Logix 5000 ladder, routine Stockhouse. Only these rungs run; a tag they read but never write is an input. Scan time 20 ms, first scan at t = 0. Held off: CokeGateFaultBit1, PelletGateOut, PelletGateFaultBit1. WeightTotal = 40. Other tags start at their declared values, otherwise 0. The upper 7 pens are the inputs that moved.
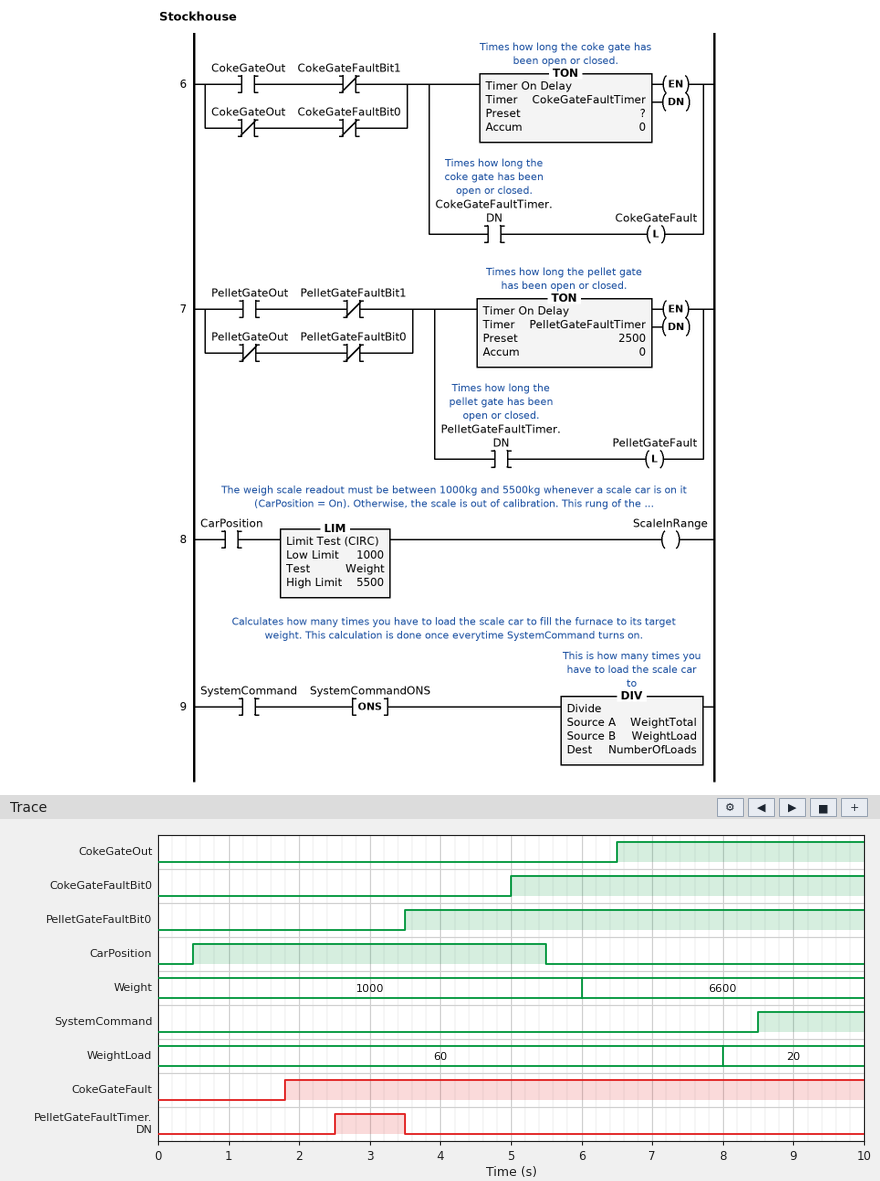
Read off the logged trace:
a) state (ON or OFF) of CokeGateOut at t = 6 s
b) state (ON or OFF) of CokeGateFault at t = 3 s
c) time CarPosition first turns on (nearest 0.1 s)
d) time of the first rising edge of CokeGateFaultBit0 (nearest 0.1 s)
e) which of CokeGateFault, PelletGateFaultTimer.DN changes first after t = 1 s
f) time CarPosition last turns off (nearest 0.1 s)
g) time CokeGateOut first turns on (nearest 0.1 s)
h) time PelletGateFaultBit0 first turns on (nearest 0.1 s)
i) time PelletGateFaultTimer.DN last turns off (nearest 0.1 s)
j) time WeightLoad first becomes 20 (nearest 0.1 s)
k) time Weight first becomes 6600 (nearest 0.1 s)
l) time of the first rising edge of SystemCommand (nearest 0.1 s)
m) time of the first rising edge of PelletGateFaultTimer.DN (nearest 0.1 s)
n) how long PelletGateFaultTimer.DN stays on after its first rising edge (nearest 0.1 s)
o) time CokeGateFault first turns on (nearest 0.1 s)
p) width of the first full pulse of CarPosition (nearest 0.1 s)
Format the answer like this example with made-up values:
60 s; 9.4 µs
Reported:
OFF; ON; 0.5 s; 5.0 s; CokeGateFault; 5.5 s; 6.5 s; 3.5 s; 3.5 s; 8.0 s; 6.0 s; 8.5 s; 2.5 s; 1.0 s; 1.8 s; 5.0 s
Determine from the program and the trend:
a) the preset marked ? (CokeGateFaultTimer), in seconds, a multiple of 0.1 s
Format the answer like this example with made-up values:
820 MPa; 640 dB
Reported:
1.8 s
